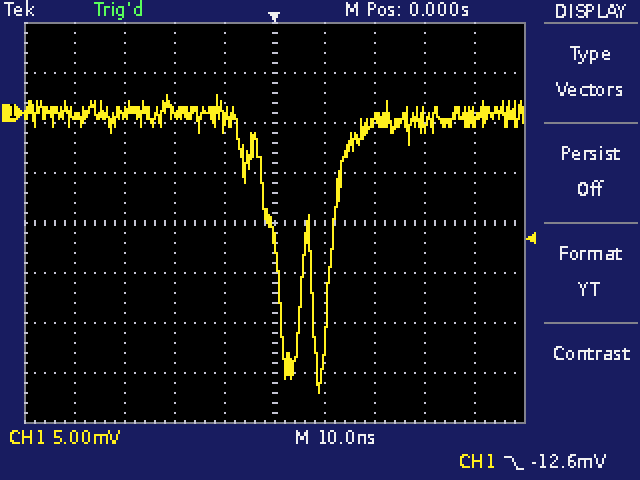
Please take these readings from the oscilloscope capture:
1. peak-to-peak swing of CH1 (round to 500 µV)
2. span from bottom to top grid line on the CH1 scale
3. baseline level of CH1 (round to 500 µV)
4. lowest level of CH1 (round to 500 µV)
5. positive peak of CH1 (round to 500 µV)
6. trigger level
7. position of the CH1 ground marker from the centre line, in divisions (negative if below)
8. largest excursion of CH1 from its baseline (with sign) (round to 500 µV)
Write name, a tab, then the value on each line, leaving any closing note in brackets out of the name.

peak-to-peak swing of CH1	30.0 mV
span from bottom to top grid line on the CH1 scale	40 mV
baseline level of CH1	-500 µV
lowest level of CH1	-28.0 mV
positive peak of CH1	2.0 mV
trigger level	-12.6 mV
position of the CH1 ground marker from the centre line, in divisions	+2.2 div
largest excursion of CH1 from its baseline (with sign)	-27.5 mV
